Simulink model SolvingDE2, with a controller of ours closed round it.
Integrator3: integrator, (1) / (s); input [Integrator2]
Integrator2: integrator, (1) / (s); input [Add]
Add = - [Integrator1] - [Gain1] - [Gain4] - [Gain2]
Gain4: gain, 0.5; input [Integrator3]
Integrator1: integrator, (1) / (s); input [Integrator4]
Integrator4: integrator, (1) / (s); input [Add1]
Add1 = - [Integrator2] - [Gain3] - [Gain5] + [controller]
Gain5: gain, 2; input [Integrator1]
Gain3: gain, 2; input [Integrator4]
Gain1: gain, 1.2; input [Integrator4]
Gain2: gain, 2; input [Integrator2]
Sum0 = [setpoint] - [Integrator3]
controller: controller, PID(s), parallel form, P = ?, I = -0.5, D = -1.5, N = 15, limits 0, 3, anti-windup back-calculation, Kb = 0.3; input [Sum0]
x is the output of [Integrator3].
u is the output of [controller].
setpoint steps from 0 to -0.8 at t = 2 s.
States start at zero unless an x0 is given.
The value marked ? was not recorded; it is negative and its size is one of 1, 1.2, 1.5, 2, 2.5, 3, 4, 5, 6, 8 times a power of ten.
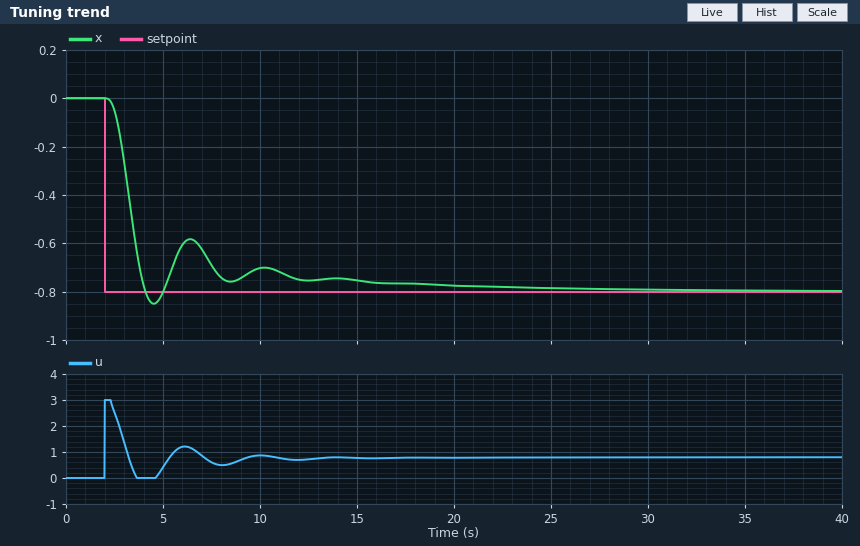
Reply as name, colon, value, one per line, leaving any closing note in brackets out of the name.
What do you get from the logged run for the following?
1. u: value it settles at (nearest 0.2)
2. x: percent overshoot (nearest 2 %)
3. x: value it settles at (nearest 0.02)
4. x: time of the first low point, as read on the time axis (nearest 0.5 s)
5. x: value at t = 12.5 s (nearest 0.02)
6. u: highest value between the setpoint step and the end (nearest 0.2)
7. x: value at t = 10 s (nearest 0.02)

u: value it settles at: 0.8
x: percent overshoot: 6 %
x: value it settles at: -0.80
x: time of the first low point, as read on the time axis: 4.5 s
x: value at t = 12.5 s: -0.76
u: highest value between the setpoint step and the end: 3.0
x: value at t = 10 s: -0.70
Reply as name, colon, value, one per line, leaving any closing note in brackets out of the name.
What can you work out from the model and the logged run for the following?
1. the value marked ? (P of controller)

the value marked ?: -4
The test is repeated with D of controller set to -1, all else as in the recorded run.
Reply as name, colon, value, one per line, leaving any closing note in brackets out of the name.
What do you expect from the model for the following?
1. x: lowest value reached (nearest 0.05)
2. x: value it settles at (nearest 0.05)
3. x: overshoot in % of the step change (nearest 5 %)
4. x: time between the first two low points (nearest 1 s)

x: lowest value reached: -0.95
x: value it settles at: -0.80
x: overshoot in % of the step change: 20 %
x: time between the first two low points: 4 s
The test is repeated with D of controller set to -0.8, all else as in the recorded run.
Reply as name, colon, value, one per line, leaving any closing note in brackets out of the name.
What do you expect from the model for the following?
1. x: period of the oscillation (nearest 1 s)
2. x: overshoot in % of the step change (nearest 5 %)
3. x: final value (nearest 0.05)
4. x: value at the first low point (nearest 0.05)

x: period of the oscillation: 4 s
x: overshoot in % of the step change: 25 %
x: final value: -0.80
x: value at the first low point: -1.00
